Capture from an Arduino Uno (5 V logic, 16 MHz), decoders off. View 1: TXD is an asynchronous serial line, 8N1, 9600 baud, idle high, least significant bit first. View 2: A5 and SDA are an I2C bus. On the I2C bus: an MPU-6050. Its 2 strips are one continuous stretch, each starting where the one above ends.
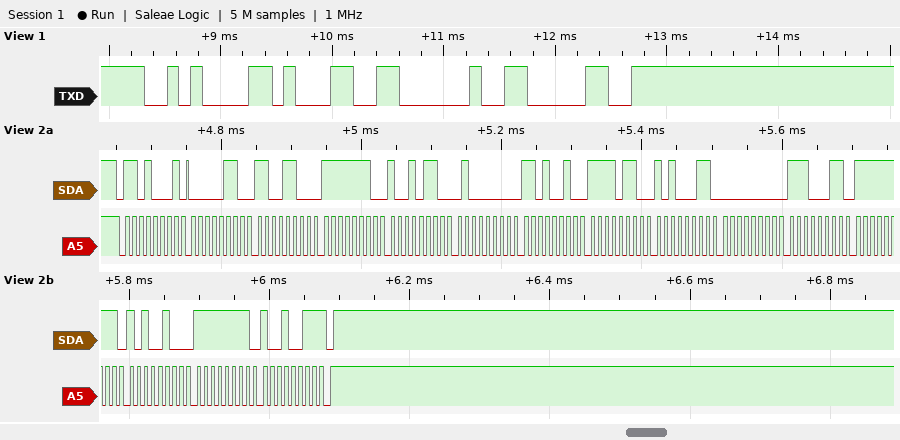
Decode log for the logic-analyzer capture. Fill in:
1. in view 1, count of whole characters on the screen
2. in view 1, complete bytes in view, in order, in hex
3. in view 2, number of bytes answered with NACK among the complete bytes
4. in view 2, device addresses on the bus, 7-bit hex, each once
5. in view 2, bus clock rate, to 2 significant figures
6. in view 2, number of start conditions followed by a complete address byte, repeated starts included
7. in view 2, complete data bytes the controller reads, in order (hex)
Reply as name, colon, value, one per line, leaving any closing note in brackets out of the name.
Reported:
in view 1, count of whole characters on the screen: 4
in view 1, complete bytes in view, in order, in hex: 0A 31 20 30
in view 2, number of bytes answered with NACK among the complete bytes: 1
in view 2, device addresses on the bus, 7-bit hex, each once: 0x68
in view 2, bus clock rate, to 2 significant figures: 100 kHz
in view 2, number of start conditions followed by a complete address byte, repeated starts included: 1
in view 2, complete data bytes the controller reads, in order: 06 CC FE 96 40 D2 F6 A3 00 E3 FF A4 FF 93
